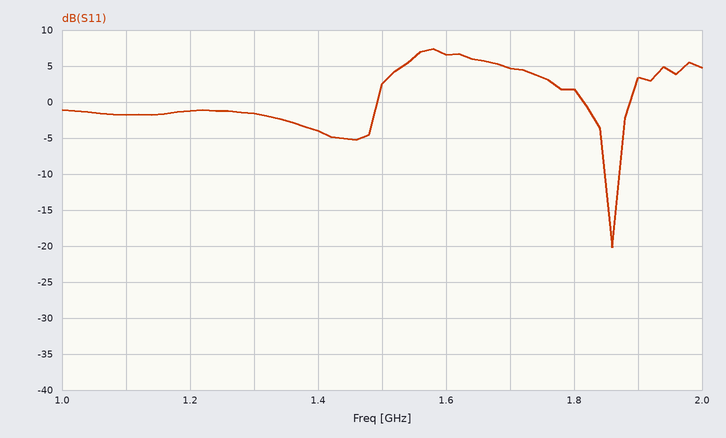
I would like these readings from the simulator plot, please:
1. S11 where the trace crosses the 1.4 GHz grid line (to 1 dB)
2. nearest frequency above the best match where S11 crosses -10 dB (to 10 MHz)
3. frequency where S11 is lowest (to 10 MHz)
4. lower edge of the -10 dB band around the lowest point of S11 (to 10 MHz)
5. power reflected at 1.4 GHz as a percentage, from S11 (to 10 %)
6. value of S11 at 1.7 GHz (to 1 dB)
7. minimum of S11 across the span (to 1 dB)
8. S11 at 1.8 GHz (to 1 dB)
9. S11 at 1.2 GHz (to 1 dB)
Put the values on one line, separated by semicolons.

-4 dB; 1.87 GHz; 1.86 GHz; 1.85 GHz; 40 %; 5 dB; -20 dB; 2 dB; -1 dB
